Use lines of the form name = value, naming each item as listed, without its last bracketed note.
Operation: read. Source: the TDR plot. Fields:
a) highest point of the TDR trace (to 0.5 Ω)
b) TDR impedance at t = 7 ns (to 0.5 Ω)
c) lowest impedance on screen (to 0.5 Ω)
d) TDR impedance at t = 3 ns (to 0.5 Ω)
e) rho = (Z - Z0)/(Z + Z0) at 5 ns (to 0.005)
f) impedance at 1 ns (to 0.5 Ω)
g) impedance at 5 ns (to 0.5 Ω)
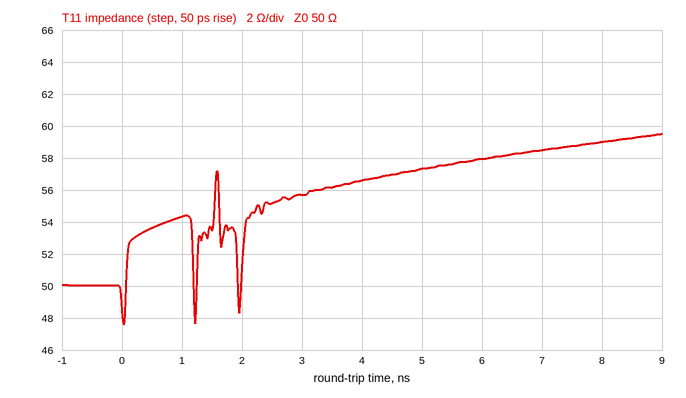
highest point of the TDR trace = 59.5 Ω
TDR impedance at t = 7 ns = 58.5 Ω
lowest impedance on screen = 47.5 Ω
TDR impedance at t = 3 ns = 55.5 Ω
rho = (Z - Z0)/(Z + Z0) at 5 ns = +0.070
impedance at 1 ns = 54.5 Ω
impedance at 5 ns = 57.5 Ω
